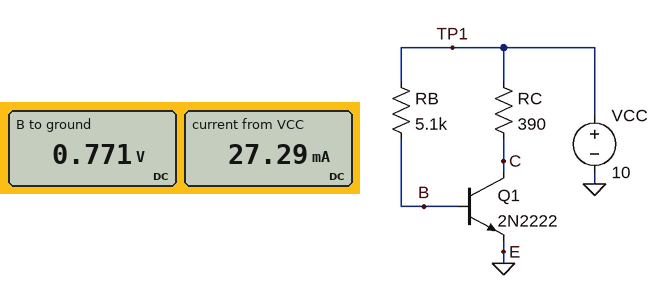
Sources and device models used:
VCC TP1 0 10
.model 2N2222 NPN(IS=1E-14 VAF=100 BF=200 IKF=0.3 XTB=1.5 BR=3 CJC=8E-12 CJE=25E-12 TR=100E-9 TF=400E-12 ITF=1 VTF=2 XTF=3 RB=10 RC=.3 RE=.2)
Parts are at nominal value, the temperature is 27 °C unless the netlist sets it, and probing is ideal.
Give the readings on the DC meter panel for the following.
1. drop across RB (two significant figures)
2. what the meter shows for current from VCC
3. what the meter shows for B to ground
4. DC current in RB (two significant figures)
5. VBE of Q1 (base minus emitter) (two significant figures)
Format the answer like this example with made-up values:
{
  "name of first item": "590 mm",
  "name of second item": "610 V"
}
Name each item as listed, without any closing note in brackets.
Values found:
{
  "drop across RB": "9.2 V",
  "what the meter shows for current from VCC": "27.29 mA",
  "what the meter shows for B to ground": "0.771 V",
  "DC current in RB": "1.8 mA",
  "VBE of Q1 (base minus emitter)": "770 mV"
}
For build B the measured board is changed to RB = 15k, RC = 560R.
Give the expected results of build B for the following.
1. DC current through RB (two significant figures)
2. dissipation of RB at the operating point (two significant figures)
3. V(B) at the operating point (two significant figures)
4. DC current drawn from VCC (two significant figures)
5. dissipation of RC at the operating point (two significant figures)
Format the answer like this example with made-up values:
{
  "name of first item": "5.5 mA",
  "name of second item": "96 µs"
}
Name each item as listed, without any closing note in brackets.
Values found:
{
  "DC current through RB": "620 µA",
  "dissipation of RB at the operating point": "5.7 mW",
  "V(B) at the operating point": "740 mV",
  "DC current drawn from VCC": "18 mA",
  "dissipation of RC at the operating point": "180 mW"
}
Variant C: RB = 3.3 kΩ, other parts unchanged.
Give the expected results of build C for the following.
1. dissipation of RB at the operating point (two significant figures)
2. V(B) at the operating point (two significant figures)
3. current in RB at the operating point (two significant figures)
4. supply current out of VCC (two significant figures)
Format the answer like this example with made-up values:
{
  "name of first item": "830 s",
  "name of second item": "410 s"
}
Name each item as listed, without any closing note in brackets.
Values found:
{
  "dissipation of RB at the operating point": "26 mW",
  "V(B) at the operating point": "780 mV",
  "current in RB at the operating point": "2.8 mA",
  "supply current out of VCC": "28 mA"
}
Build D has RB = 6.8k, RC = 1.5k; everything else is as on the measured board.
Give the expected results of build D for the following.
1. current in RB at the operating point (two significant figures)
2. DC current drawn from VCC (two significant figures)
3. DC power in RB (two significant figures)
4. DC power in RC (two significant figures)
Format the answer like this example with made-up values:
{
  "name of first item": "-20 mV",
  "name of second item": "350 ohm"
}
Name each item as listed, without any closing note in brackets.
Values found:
{
  "current in RB at the operating point": "1.4 mA",
  "DC current drawn from VCC": "8.0 mA",
  "DC power in RB": "13 mW",
  "DC power in RC": "66 mW"
}
